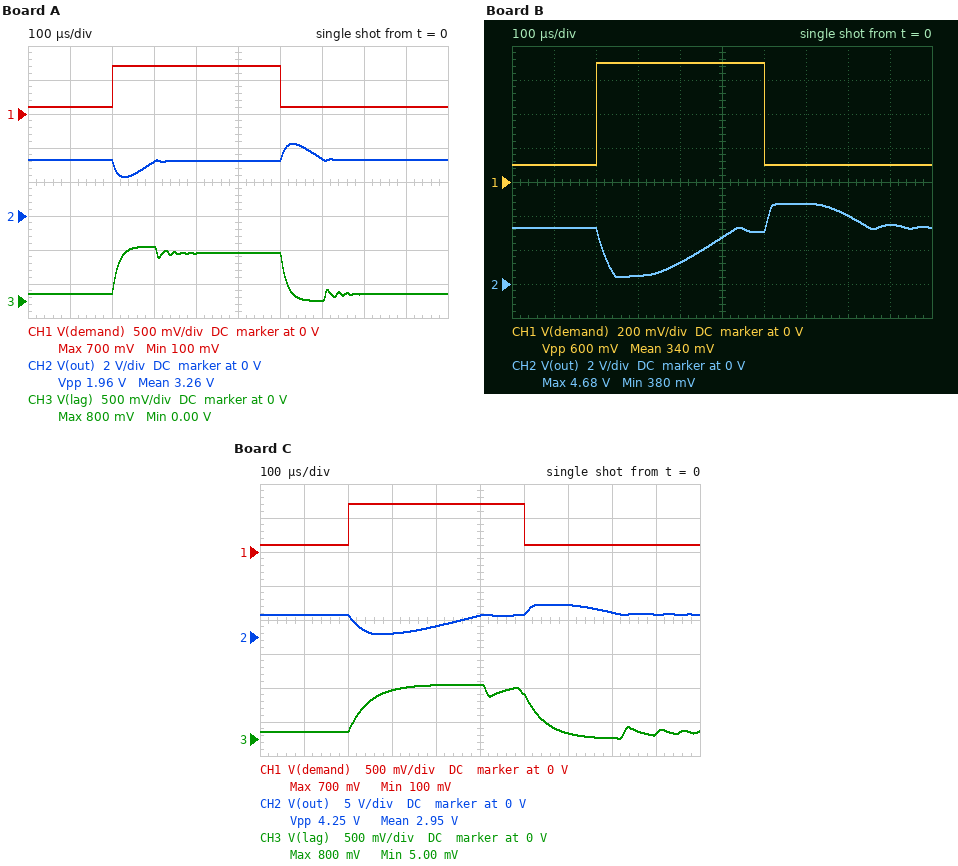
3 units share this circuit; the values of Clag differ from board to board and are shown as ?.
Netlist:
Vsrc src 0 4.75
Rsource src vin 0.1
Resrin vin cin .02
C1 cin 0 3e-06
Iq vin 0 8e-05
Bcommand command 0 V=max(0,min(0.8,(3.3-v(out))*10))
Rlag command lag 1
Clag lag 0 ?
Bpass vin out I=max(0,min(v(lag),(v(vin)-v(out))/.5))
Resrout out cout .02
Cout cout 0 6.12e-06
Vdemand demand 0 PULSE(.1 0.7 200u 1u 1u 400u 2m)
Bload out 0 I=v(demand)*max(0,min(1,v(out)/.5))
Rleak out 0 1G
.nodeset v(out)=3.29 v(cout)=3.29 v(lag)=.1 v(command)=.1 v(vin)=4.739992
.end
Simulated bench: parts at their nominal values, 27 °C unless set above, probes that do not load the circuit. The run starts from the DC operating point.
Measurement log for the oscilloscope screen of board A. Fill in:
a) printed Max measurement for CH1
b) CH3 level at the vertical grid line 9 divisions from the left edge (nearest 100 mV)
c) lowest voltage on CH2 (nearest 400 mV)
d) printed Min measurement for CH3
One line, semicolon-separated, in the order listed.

700 mV; 100 mV; 2.4 V; 0.00 V
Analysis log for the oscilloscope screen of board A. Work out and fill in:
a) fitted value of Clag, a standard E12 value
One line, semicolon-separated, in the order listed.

15 µF
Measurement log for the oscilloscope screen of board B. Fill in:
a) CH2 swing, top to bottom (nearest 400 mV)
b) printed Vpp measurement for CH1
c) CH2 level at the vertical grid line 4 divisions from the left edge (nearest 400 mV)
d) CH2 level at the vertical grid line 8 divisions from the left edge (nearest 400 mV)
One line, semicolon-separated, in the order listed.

4.4 V; 600 mV; 1.2 V; 4.0 V
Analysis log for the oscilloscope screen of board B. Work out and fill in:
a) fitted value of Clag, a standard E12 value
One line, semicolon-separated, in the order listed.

56 µF
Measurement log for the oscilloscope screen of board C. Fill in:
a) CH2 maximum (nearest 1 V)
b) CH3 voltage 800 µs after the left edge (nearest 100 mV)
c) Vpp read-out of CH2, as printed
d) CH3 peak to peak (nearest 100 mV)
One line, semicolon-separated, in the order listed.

5 V; 0 V; 4.25 V; 800 mV
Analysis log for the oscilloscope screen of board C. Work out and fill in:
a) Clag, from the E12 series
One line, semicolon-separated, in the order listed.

47 µF
